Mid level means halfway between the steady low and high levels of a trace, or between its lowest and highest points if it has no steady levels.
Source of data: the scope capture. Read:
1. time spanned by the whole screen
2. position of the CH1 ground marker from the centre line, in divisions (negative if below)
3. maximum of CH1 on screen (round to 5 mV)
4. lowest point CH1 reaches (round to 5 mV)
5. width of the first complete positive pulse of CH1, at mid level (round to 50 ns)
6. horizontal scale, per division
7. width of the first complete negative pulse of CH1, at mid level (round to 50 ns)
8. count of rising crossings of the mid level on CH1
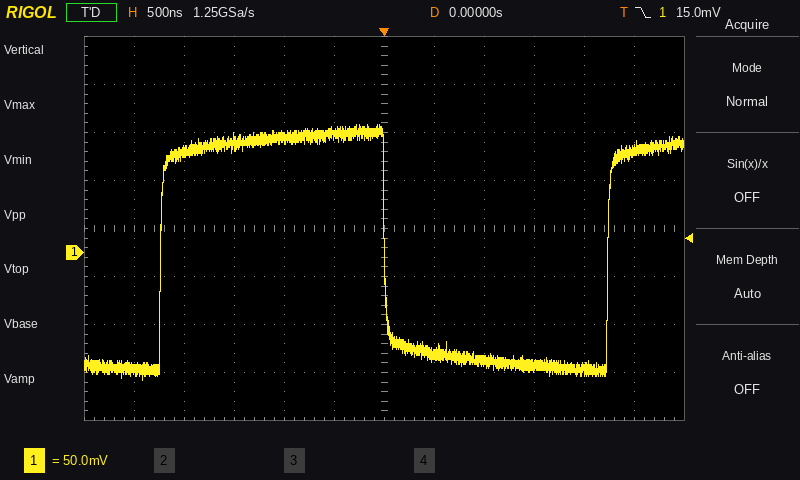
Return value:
6 µs
-0.5 div
135 mV
-135 mV
2.25 µs
500 ns
2.25 µs
2
